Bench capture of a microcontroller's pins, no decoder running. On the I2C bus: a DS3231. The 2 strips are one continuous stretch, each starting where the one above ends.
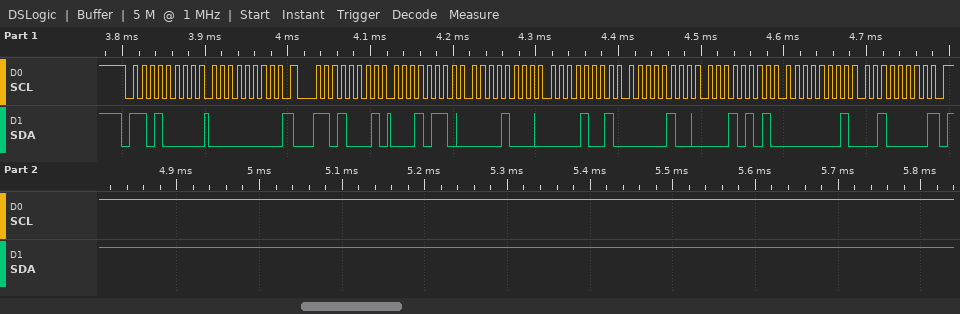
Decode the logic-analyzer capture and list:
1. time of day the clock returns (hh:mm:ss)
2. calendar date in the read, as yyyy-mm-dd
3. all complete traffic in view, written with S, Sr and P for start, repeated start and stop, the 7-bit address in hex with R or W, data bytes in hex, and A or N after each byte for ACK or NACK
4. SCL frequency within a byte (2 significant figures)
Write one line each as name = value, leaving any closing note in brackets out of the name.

time of day the clock returns = 09:08:16
calendar date in the read, as yyyy-mm-dd = 2020-01-15
all complete traffic in view, written with S, Sr and P for start, repeated start and stop, the 7-bit address in hex with R or W, data bytes in hex, and A or N after each byte for ACK or NACK = S 68W A 00 A Sr 68R A 16 A 08 A 09 A 04 A 15 A 01 A 20 N P
SCL frequency within a byte = 100 kHz
